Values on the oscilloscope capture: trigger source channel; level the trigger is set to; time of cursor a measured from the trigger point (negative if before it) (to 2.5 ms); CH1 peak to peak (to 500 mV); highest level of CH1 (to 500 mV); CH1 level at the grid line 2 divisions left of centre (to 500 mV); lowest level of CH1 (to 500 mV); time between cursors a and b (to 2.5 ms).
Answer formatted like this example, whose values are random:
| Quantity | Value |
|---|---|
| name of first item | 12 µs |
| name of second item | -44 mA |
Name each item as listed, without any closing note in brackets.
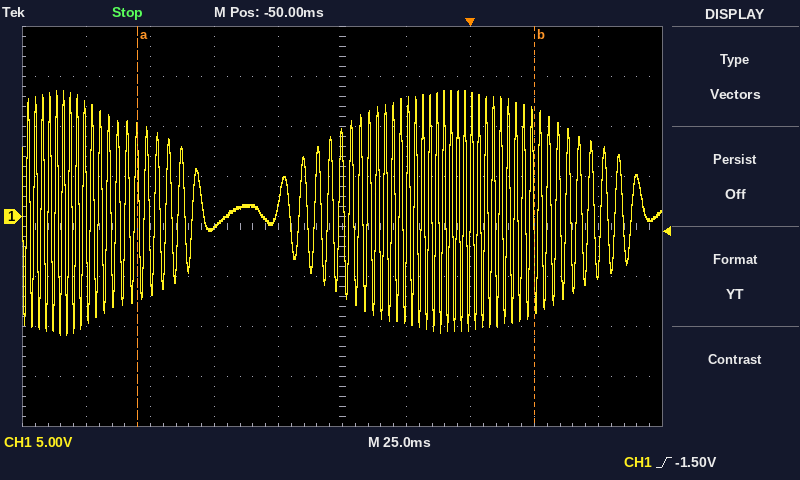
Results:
| Quantity | Value |
|---|---|
| trigger source channel | CH1 |
| level the trigger is set to | -1.50 V |
| time of cursor a measured from the trigger point (negative if before it) | -130.0 ms |
| CH1 peak to peak | 24.5 V |
| highest level of CH1 | 12.5 V |
| CH1 level at the grid line 2 divisions left of centre | -1.0 V |
| lowest level of CH1 | -12.0 V |
| time between cursors a and b | 155.0 ms |
